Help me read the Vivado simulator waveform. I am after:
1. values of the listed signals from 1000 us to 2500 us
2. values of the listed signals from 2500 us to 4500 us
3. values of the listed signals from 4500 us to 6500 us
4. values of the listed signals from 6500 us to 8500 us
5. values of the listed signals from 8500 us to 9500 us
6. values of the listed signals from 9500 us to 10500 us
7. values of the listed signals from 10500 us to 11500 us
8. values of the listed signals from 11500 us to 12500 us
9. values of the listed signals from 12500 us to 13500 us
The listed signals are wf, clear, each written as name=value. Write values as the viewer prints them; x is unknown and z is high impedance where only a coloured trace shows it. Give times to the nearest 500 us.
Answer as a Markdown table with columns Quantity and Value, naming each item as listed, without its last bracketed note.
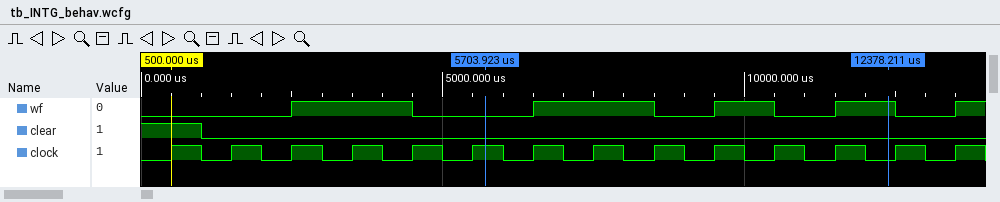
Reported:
| Quantity | Value |
|---|---|
| values of the listed signals from 1000 us to 2500 us | wf=0, clear=0 |
| values of the listed signals from 2500 us to 4500 us | wf=1, clear=0 |
| values of the listed signals from 4500 us to 6500 us | wf=0, clear=0 |
| values of the listed signals from 6500 us to 8500 us | wf=1, clear=0 |
| values of the listed signals from 8500 us to 9500 us | wf=0, clear=0 |
| values of the listed signals from 9500 us to 10500 us | wf=1, clear=0 |
| values of the listed signals from 10500 us to 11500 us | wf=0, clear=0 |
| values of the listed signals from 11500 us to 12500 us | wf=1, clear=0 |
| values of the listed signals from 12500 us to 13500 us | wf=0, clear=0 |
